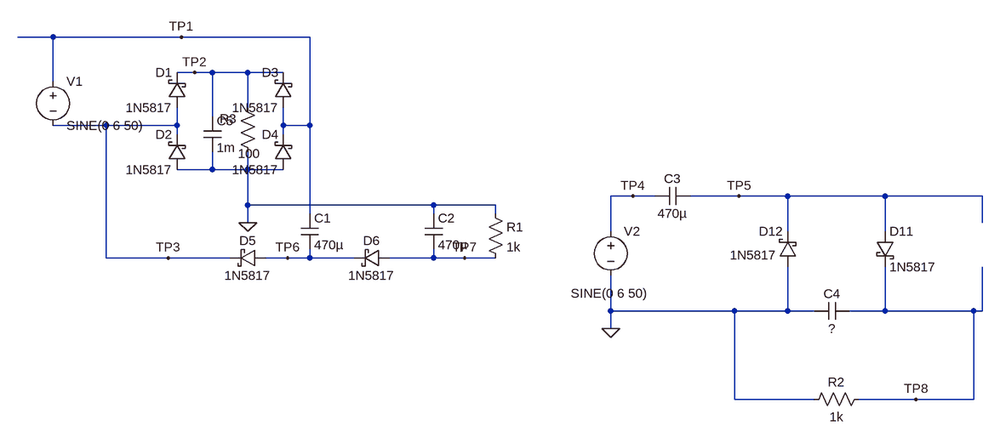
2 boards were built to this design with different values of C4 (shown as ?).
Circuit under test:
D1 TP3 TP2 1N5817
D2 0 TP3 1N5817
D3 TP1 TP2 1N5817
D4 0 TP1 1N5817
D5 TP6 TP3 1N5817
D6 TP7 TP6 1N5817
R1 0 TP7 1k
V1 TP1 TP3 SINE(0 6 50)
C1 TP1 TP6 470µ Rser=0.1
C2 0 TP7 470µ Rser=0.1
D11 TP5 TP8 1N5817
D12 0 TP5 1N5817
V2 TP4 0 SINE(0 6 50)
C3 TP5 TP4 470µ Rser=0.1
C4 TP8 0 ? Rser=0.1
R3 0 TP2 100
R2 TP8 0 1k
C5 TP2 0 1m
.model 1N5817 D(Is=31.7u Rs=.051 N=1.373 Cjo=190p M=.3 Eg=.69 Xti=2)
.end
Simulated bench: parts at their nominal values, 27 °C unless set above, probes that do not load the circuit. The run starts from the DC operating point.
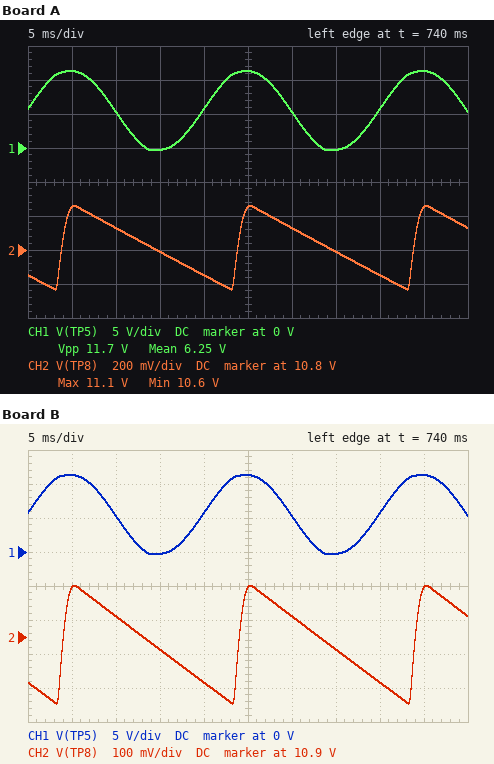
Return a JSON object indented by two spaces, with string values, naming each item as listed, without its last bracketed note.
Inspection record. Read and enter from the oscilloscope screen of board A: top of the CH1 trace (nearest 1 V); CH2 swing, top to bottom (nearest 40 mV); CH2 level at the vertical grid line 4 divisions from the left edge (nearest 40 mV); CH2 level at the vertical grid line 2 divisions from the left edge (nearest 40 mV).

{
  "top of the CH1 trace": "11 V",
  "CH2 swing, top to bottom": "480 mV",
  "CH2 level at the vertical grid line 4 divisions from the left edge": "10.64 V",
  "CH2 level at the vertical grid line 2 divisions from the left edge": "10.92 V"
}
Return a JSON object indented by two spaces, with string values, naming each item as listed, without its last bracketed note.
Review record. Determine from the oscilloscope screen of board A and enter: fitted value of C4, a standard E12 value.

{
  "fitted value of C4, a standard E12 value": "390 µF"
}
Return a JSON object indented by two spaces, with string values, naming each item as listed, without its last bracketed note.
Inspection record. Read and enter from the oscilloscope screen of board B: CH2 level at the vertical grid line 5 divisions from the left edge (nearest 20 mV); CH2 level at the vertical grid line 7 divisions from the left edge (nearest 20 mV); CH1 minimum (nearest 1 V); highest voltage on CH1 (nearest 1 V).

{
  "CH2 level at the vertical grid line 5 divisions from the left edge": "11.04 V",
  "CH2 level at the vertical grid line 7 divisions from the left edge": "10.86 V",
  "CH1 minimum": "0 V",
  "highest voltage on CH1": "11 V"
}
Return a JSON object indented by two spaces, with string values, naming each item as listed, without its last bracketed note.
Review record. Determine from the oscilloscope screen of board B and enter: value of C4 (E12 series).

{
  "value of C4": "560 µF"
}
